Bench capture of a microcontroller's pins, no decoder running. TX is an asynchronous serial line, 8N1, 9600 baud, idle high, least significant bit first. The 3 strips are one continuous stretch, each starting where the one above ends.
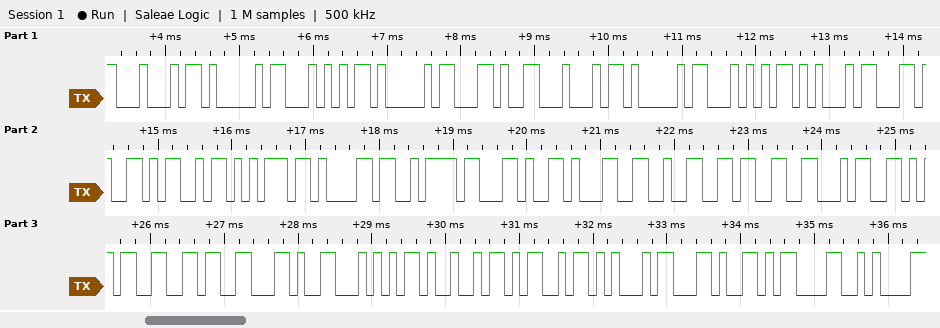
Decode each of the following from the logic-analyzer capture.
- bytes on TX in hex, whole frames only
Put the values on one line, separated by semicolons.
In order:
44 41 54 41 2C 44 41 54 45 2C 4D 75 61 7A 2C 31 32 33 34 35 36 2C 54 49 4D 45 2C 0D 0A
